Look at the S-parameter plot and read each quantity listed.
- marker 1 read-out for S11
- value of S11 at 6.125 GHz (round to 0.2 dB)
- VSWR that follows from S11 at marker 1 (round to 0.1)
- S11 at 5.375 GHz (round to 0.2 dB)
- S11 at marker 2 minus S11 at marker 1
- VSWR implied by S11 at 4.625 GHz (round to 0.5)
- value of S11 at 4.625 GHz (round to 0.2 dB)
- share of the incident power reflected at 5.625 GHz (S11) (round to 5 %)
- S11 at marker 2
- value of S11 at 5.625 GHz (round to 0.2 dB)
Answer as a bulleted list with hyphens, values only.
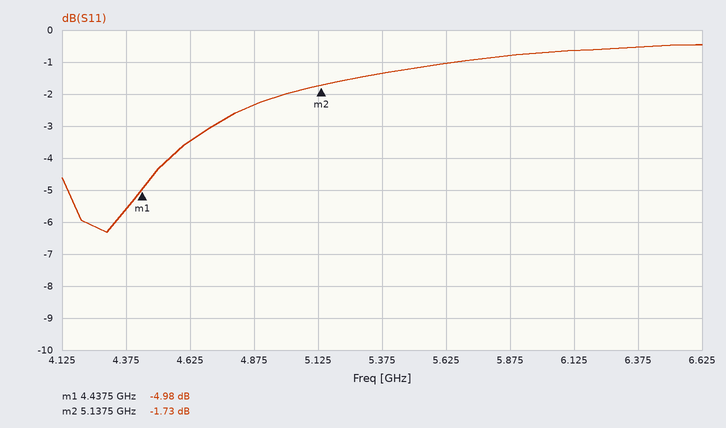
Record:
- -4.98 dB
- -0.6 dB
- 3.6
- -1.4 dB
- 3.25 dB
- 5.0
- -3.4 dB
- 80 %
- -1.73 dB
- -1.0 dB
